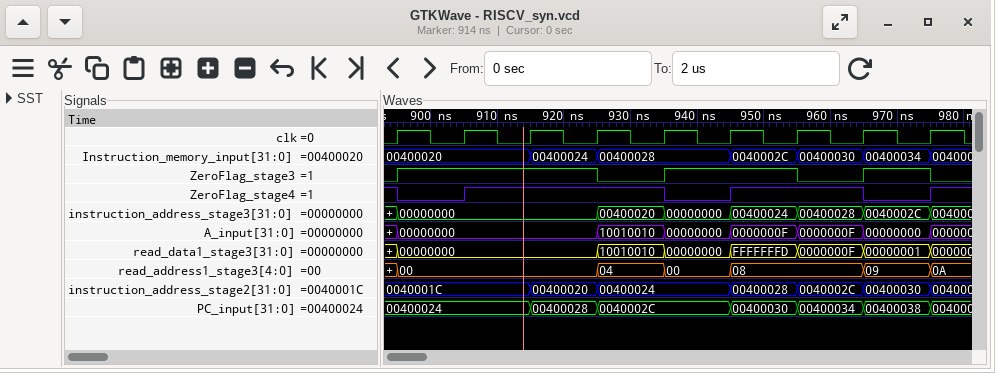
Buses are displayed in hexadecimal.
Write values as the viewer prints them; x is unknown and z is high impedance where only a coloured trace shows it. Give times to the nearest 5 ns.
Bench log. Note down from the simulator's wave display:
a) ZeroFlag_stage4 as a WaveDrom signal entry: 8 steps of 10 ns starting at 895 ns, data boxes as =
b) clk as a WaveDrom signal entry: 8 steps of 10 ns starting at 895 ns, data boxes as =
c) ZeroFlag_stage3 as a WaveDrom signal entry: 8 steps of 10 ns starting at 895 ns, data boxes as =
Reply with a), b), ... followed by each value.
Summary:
a) {name: 'ZeroFlag_stage4', wave: '01..01.0'}
b) {name: 'clk', wave: 'p.......'}
c) {name: 'ZeroFlag_stage3', wave: '1..01.01'}
